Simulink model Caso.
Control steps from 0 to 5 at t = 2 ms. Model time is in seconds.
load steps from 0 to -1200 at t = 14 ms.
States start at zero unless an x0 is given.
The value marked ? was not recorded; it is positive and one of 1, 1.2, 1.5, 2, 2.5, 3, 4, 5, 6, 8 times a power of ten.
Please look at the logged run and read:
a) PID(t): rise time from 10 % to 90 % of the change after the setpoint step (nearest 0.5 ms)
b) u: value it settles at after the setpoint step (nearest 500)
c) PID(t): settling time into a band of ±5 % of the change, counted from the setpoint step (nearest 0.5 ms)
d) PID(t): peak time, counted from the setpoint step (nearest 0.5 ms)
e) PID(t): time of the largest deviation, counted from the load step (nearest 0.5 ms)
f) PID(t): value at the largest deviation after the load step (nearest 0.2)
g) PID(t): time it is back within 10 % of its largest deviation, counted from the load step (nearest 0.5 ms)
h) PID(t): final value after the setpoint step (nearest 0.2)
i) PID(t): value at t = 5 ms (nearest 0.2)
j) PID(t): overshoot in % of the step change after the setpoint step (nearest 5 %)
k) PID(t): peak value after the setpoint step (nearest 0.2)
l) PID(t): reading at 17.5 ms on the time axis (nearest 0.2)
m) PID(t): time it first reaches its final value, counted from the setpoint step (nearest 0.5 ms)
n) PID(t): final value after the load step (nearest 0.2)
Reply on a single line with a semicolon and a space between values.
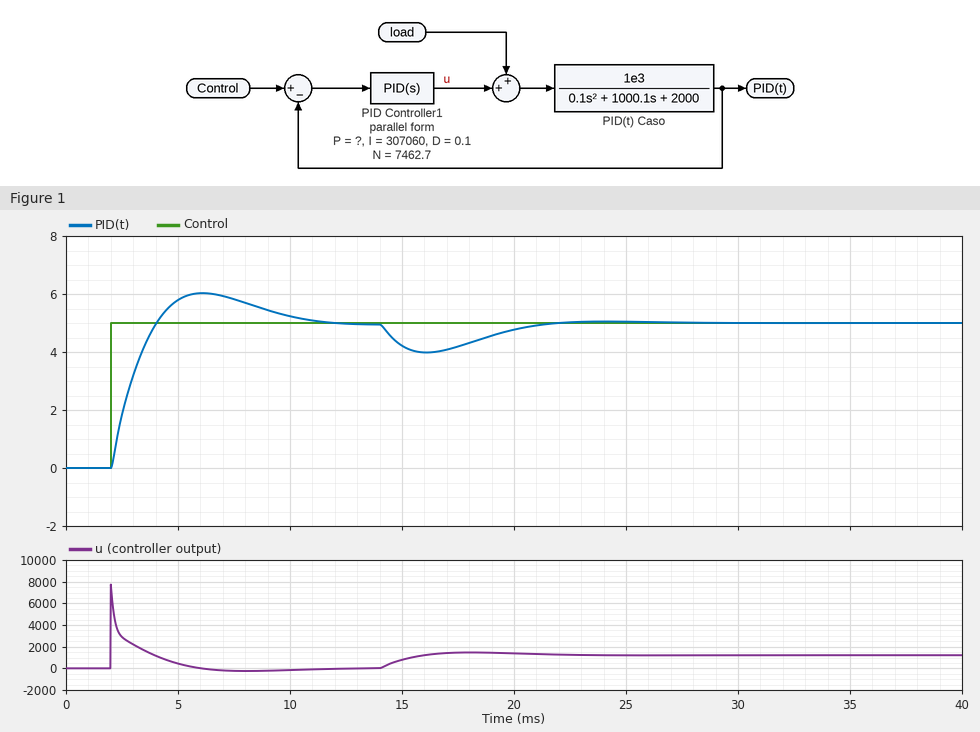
1.5 ms; 0; 8.0 ms; 4.0 ms; 2.0 ms; 4.0; 7.0 ms; 5.0; 5.8; 20 %; 6.0; 4.2; 2.0 ms; 5.0
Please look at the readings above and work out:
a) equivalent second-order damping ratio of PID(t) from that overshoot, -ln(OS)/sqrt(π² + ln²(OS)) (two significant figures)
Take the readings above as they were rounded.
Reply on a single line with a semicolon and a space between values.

0.46
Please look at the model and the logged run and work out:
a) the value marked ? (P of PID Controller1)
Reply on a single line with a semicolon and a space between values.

800
